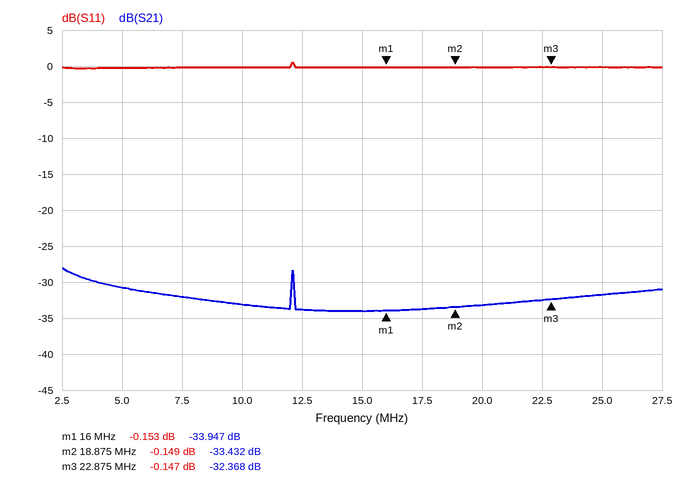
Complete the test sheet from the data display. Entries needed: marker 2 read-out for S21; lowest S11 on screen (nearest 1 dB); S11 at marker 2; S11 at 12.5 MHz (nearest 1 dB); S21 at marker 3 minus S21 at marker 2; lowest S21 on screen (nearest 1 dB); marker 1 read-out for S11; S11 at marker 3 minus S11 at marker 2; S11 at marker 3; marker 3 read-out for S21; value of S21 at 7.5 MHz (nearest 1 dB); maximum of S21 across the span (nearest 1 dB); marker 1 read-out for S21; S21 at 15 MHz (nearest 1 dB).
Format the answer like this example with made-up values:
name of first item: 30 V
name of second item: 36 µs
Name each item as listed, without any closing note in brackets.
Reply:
marker 2 read-out for S21: -33.432 dB
lowest S11 on screen: 0 dB
S11 at marker 2: -0.149 dB
S11 at 12.5 MHz: 0 dB
S21 at marker 3 minus S21 at marker 2: 1.064 dB
lowest S21 on screen: -34 dB
marker 1 read-out for S11: -0.153 dB
S11 at marker 3 minus S11 at marker 2: 0.002 dB
S11 at marker 3: -0.147 dB
marker 3 read-out for S21: -32.368 dB
value of S21 at 7.5 MHz: -32 dB
maximum of S21 across the span: -28 dB
marker 1 read-out for S21: -33.947 dB
S21 at 15 MHz: -34 dB
